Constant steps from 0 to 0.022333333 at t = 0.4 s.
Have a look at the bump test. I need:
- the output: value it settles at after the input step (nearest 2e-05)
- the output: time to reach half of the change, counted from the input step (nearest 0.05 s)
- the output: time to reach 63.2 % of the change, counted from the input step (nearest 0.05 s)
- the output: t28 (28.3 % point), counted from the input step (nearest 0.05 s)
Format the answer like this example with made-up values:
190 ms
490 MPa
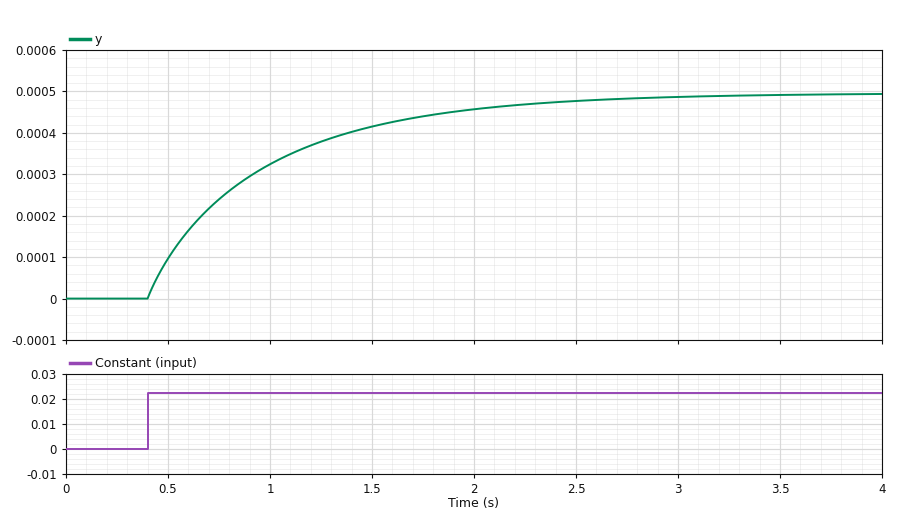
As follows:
0.00050
0.35 s
0.55 s
0.15 s
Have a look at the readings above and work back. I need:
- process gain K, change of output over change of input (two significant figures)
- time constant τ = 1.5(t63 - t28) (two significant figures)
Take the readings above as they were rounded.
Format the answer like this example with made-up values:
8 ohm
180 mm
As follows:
0.022
0.60 s
